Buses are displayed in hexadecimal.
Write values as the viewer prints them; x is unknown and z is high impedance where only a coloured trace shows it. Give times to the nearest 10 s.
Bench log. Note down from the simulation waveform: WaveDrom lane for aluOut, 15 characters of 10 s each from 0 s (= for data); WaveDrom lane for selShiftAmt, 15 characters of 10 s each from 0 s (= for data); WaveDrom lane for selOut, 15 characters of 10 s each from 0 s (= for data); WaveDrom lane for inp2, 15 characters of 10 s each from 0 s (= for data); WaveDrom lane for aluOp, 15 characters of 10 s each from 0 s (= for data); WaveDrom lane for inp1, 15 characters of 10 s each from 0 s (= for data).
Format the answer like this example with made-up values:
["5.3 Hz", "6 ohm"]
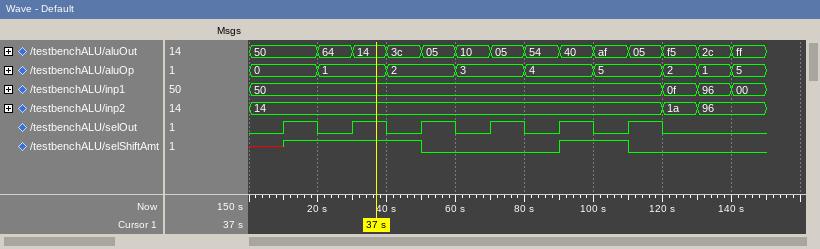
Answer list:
["{name: 'aluOut', wave: '=.=============', data: '50 64 14 3c 05 10 05 54 40 af 05 f5 2c ff'}", "{name: 'selShiftAmt', wave: 'x1...0...1.0...'}", "{name: 'selOut', wave: '0101010101010..'}", "{name: 'inp2', wave: '=...........==.', data: '14 1a 96'}", "{name: 'aluOp', wave: '=.=.=.=.=.=.===', data: '0 1 2 3 4 5 2 1 5'}", "{name: 'inp1', wave: '=...........===', data: '50 0f 96 00'}"]
